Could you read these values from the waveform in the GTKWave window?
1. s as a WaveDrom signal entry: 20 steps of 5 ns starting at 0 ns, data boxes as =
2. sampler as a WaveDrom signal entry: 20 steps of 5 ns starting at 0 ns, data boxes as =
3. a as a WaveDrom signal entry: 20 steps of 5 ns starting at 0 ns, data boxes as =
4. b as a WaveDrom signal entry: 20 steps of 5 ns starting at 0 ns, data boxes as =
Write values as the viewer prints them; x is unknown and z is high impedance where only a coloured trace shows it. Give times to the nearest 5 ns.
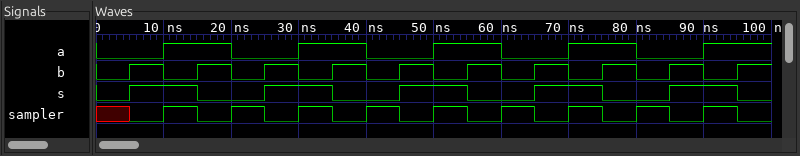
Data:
{name: 's', wave: '01.0.1.0.1.0.1.0.1.0'}
{name: 'sampler', wave: 'x0101010101010101010'}
{name: 'a', wave: '0.1.0.1.0.1.0.1.0.1.'}
{name: 'b', wave: '01010101010101010101'}
